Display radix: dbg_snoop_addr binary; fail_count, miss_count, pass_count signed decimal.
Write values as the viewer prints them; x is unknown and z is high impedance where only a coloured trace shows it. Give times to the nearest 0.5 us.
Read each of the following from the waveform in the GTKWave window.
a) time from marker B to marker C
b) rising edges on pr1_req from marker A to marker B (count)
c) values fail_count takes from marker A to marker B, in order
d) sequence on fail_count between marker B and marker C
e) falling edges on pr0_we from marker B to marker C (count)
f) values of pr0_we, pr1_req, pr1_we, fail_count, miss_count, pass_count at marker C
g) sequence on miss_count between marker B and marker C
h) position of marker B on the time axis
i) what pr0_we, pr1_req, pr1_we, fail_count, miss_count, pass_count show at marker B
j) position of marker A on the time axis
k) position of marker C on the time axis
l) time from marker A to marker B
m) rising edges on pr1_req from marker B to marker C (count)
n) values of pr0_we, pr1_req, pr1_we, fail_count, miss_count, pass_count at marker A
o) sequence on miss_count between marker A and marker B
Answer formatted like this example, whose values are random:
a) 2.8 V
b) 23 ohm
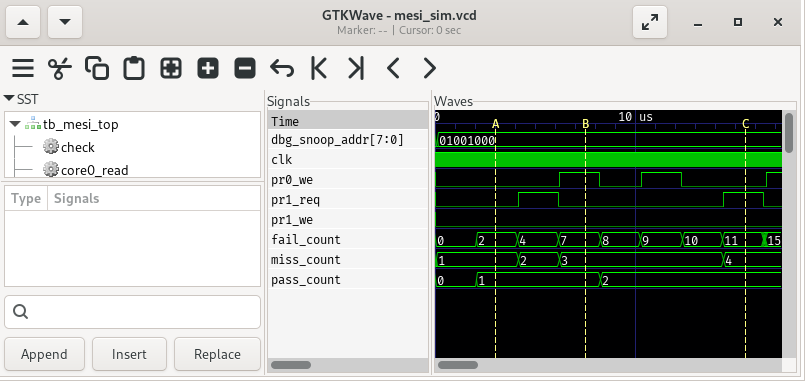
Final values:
a) 8 us
b) 1
c) 2, 4, 7
d) 7, 8, 9, 10, 11
e) 2
f) pr0_we=0, pr1_req=1, pr1_we=0, fail_count=11, miss_count=4, pass_count=2
g) 3, 4
h) 7.5 us
i) pr0_we=1, pr1_req=0, pr1_we=0, fail_count=7, miss_count=3, pass_count=1
j) 3 us
k) 15.5 us
l) 4.5 us
m) 1
n) pr0_we=0, pr1_req=0, pr1_we=0, fail_count=2, miss_count=1, pass_count=1
o) 1, 2, 3
